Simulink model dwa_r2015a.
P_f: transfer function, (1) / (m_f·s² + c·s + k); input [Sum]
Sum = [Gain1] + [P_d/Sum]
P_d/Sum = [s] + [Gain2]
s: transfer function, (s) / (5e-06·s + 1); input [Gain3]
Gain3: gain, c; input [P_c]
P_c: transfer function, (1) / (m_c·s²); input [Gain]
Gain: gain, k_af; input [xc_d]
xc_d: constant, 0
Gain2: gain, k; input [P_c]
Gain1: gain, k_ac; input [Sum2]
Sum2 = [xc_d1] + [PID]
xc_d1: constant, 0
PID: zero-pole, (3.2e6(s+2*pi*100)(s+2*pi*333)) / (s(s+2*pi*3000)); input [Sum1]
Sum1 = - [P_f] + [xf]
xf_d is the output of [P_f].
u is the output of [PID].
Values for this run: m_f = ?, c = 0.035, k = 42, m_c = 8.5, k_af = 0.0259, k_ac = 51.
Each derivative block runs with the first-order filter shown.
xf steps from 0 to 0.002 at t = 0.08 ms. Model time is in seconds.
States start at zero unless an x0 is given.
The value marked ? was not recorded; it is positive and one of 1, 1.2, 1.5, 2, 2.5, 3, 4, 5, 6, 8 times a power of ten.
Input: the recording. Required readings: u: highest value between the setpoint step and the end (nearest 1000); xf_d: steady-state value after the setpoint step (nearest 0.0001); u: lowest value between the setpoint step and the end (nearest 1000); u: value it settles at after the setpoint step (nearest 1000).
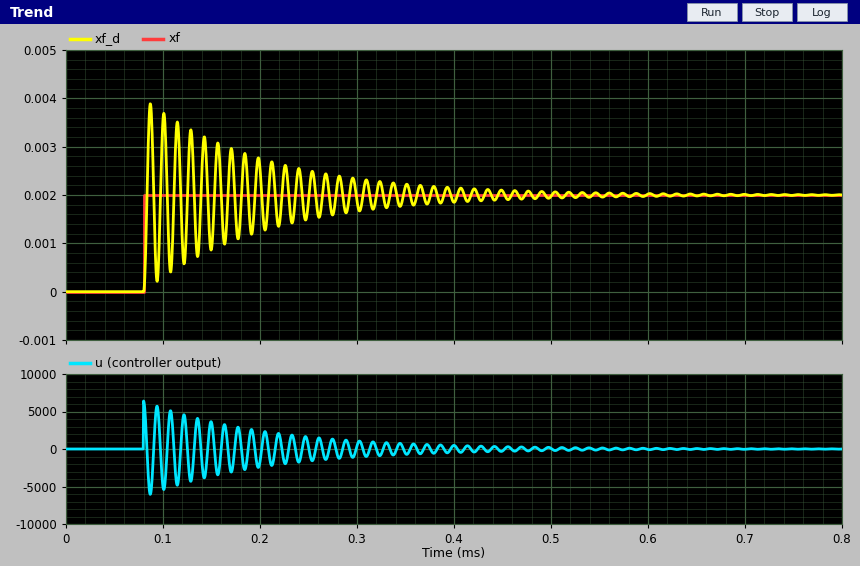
6000
0.0020
-6000
0
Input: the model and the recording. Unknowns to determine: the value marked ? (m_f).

0.0008
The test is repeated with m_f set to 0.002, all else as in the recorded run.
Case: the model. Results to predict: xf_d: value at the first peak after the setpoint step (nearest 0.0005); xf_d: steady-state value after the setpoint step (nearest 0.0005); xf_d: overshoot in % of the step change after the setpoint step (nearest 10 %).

0.0040
0.0020
90 %
